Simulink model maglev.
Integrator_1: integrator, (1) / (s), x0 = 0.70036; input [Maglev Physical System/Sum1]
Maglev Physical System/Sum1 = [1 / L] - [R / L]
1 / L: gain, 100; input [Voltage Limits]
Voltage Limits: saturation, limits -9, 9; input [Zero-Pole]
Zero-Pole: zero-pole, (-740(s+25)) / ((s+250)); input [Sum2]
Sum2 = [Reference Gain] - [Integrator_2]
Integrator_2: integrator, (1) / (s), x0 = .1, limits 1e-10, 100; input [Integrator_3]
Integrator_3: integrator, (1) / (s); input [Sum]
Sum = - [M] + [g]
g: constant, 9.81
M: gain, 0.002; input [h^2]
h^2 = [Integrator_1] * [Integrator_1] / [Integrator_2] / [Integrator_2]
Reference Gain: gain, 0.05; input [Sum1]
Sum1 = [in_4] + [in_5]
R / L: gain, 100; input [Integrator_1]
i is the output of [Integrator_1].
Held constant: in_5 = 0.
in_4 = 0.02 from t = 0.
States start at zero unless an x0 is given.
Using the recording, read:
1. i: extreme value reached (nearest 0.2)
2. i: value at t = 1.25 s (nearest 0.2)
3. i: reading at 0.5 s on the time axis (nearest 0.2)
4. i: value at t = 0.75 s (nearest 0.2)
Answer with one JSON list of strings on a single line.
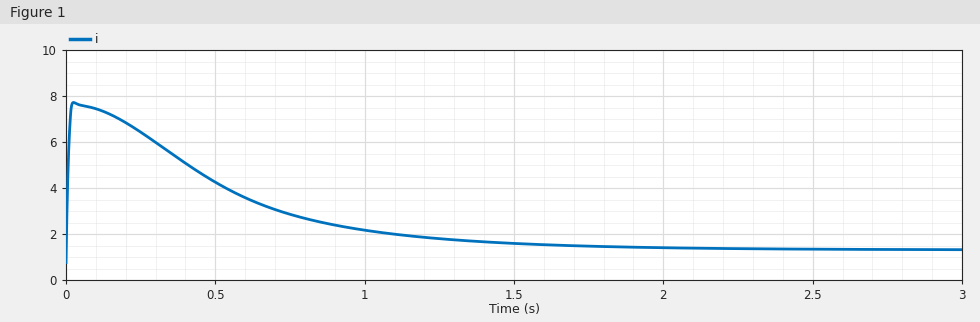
["7.8", "1.8", "4.2", "2.8"]
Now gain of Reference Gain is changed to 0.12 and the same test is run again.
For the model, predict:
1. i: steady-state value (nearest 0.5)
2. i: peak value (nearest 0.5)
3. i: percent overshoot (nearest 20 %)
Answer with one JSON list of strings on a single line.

["3.0", "7.5", "180 %"]
